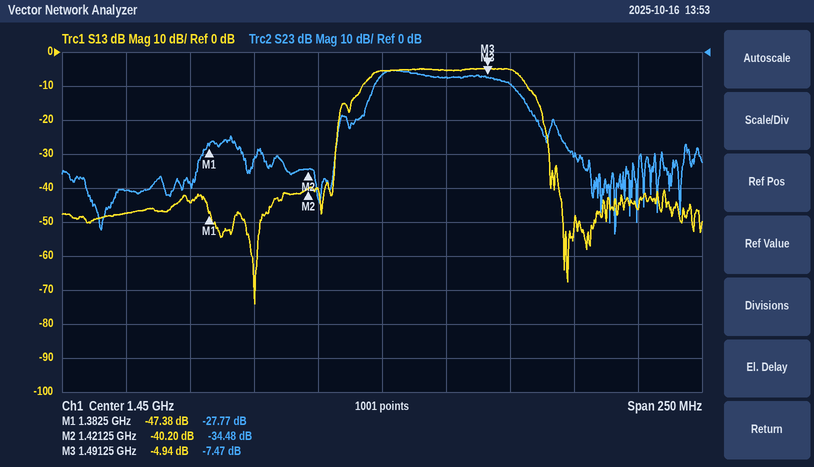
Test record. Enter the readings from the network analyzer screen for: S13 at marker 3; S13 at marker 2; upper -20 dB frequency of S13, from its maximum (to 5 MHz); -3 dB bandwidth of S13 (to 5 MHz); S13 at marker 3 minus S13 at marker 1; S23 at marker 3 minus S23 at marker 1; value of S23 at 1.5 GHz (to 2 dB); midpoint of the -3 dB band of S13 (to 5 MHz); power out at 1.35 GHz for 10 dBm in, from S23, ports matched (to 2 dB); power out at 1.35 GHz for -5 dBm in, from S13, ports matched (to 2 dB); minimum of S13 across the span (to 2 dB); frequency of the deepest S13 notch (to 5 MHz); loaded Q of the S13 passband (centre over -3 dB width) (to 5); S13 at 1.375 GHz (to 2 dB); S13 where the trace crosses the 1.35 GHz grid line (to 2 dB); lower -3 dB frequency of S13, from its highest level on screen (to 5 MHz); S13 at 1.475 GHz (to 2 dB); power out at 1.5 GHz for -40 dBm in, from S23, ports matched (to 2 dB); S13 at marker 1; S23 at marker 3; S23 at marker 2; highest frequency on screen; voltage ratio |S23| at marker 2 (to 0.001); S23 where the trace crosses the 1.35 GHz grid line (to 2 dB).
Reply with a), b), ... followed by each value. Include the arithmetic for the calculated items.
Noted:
a) -4.94 dB
b) -40.20 dB
c) 1.515 GHz
d) 1.505 GHz − 1.445 GHz = 60 MHz
e) -4.94 − (-47.38) = 42.44 dB
f) -7.47 − (-27.77) = 20.30 dB
g) -10 dB
h) 1.475 GHz
i) 10 dBm + (-40 dB) = -30 dBm
j) -5 dBm + (-48 dB) = -52 dBm
k) -74 dB
l) 1.400 GHz
m) 1.475 GHz / 60 MHz ≈ 25
n) -44 dB
o) -48 dB
p) 1.445 GHz
q) -6 dB
r) -40 dBm + (-10 dB) = -50 dBm
s) -47.38 dB
t) -7.47 dB
u) -34.48 dB
v) 1.575 GHz
w) 10^(-34.48/20) ≈ 0.019
x) -40 dB
